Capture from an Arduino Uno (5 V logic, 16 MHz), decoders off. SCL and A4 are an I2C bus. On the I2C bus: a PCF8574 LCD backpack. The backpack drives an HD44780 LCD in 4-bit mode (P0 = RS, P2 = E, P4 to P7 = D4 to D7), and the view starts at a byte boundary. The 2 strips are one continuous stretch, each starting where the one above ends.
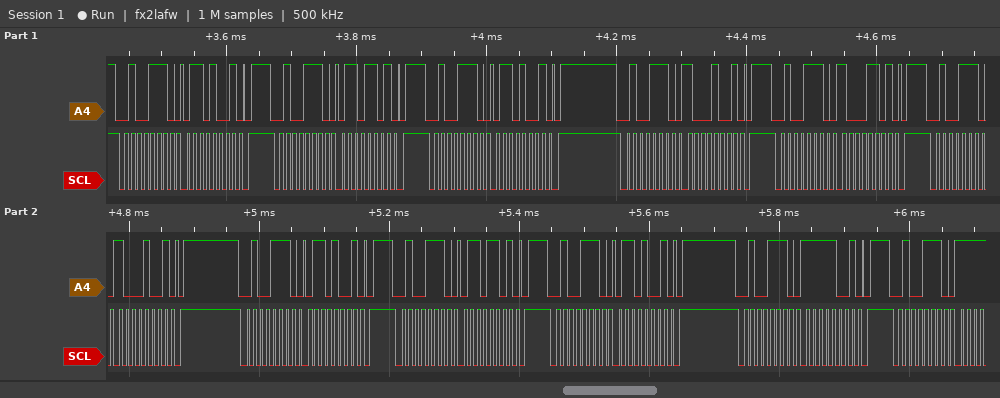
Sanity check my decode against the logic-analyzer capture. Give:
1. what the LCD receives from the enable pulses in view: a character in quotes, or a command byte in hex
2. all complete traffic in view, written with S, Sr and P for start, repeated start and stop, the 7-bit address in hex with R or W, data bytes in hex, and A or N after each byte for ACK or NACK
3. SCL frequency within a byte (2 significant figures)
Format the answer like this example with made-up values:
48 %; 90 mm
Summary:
'h'; S 27W A 69 A P S 27W A 6D A P S 27W A 69 A P S 27W A 89 A P S 27W A 8D A P S 27W A 89 A P S 27W A 69 A P S 27W A 6D A P S 27W A 69 A P S 27W A F9 A P S 27W A; 100 kHz
